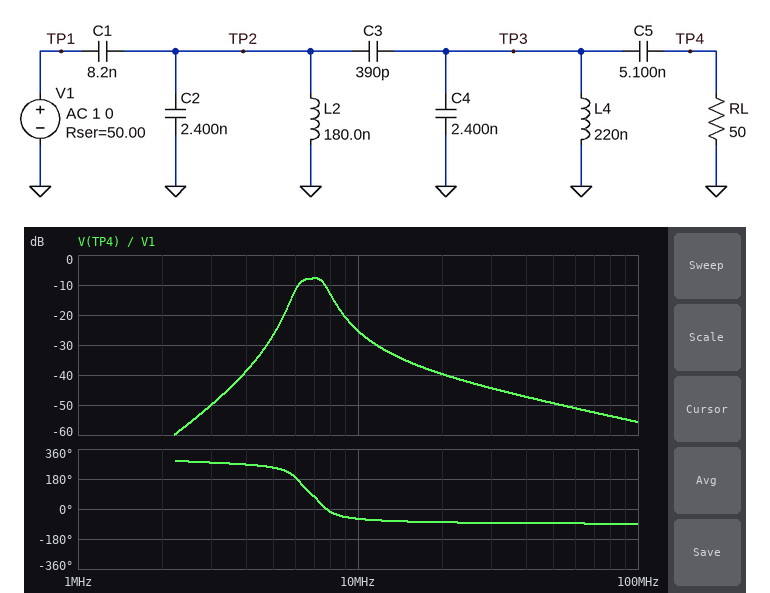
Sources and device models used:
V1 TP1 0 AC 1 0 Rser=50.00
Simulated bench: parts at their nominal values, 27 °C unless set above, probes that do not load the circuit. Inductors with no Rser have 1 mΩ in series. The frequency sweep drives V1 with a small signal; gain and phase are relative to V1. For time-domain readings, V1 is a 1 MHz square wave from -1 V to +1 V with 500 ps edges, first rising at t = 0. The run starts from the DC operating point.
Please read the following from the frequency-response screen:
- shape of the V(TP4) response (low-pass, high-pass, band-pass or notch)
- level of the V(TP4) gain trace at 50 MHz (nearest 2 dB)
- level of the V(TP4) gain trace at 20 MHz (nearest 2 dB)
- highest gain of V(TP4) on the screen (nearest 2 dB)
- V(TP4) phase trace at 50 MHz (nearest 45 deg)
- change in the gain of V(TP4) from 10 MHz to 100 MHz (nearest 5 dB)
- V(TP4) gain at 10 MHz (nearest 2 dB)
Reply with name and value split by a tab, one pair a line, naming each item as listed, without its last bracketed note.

shape of the V(TP4) response	band-pass
level of the V(TP4) gain trace at 50 MHz	-50 dB
level of the V(TP4) gain trace at 20 MHz	-40 dB
highest gain of V(TP4) on the screen	-8 dB
V(TP4) phase trace at 50 MHz	-90 deg
change in the gain of V(TP4) from 10 MHz to 100 MHz	-30 dB
V(TP4) gain at 10 MHz	-26 dB
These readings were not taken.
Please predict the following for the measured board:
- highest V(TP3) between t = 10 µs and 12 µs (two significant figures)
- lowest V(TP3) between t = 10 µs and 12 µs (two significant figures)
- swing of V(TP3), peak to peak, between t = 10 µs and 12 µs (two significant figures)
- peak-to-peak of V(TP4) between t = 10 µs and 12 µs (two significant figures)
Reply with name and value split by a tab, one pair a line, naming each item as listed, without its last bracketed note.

highest V(TP3) between t = 10 µs and 12 µs	94 mV
lowest V(TP3) between t = 10 µs and 12 µs	-94 mV
swing of V(TP3), peak to peak, between t = 10 µs and 12 µs	190 mV
peak-to-peak of V(TP4) between t = 10 µs and 12 µs	190 mV
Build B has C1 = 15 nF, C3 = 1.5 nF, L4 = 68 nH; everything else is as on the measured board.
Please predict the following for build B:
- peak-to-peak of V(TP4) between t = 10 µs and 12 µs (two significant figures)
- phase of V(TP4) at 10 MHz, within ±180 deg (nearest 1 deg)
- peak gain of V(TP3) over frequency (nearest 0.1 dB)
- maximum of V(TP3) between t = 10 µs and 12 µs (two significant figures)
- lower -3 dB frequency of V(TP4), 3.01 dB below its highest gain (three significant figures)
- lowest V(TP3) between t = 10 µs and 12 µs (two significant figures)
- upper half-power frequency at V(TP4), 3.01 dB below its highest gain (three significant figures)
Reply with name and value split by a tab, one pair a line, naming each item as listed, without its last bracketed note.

peak-to-peak of V(TP4) between t = 10 µs and 12 µs	200 mV
phase of V(TP4) at 10 MHz, within ±180 deg	70 deg
peak gain of V(TP3) over frequency	-7.5 dB
maximum of V(TP3) between t = 10 µs and 12 µs	100 mV
lower -3 dB frequency of V(TP4), 3.01 dB below its highest gain	10.3 MHz
lowest V(TP3) between t = 10 µs and 12 µs	-100 mV
upper half-power frequency at V(TP4), 3.01 dB below its highest gain	11.5 MHz
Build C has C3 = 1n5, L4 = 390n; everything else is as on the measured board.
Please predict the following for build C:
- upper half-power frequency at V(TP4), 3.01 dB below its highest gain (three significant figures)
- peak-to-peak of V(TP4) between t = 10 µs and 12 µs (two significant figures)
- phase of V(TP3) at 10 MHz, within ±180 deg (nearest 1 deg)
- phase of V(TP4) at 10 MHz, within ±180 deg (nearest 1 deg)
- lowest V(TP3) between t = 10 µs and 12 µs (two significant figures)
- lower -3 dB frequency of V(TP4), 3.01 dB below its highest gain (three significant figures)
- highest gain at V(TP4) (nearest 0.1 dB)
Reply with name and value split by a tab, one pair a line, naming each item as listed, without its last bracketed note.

upper half-power frequency at V(TP4), 3.01 dB below its highest gain	7.35 MHz
peak-to-peak of V(TP4) between t = 10 µs and 12 µs	270 mV
phase of V(TP3) at 10 MHz, within ±180 deg	-70 deg
phase of V(TP4) at 10 MHz, within ±180 deg	-67 deg
lowest V(TP3) between t = 10 µs and 12 µs	-140 mV
lower -3 dB frequency of V(TP4), 3.01 dB below its highest gain	6.09 MHz
highest gain at V(TP4)	-7.2 dB
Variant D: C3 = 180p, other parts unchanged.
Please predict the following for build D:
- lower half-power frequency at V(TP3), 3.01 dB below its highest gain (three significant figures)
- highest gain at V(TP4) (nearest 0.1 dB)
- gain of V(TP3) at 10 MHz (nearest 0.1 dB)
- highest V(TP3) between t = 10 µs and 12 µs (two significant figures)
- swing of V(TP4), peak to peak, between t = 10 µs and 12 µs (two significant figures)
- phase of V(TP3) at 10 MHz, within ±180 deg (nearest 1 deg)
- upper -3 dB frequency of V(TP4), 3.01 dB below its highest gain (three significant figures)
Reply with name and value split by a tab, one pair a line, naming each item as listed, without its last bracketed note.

lower half-power frequency at V(TP3), 3.01 dB below its highest gain	6.46 MHz
highest gain at V(TP4)	-11.5 dB
gain of V(TP3) at 10 MHz	-29.9 dB
highest V(TP3) between t = 10 µs and 12 µs	59 mV
swing of V(TP4), peak to peak, between t = 10 µs and 12 µs	120 mV
phase of V(TP3) at 10 MHz, within ±180 deg	-60 deg
upper -3 dB frequency of V(TP4), 3.01 dB below its highest gain	7.75 MHz
